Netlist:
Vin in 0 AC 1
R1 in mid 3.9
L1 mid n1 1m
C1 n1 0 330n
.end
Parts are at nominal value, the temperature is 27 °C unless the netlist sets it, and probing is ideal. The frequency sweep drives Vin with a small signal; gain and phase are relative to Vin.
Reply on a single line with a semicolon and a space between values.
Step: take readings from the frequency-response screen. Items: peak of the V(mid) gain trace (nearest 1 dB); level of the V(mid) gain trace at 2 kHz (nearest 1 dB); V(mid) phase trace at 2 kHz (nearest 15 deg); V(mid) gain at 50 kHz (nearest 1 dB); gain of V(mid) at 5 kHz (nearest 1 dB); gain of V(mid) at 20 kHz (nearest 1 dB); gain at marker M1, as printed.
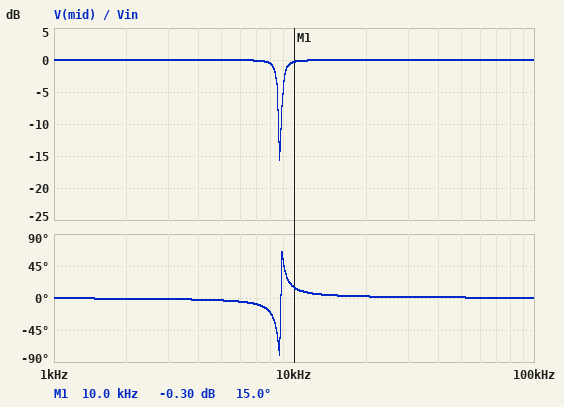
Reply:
0 dB; 0 dB; 0 deg; 0 dB; 0 dB; 0 dB; -0.30 dB
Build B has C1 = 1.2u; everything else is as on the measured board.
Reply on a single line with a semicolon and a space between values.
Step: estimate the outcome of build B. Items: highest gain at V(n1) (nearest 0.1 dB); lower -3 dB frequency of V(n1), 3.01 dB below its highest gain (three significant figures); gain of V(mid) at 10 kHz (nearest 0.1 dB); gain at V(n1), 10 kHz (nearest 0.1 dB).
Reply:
17.4 dB; 4.25 kHz; 0 dB; -11.5 dB
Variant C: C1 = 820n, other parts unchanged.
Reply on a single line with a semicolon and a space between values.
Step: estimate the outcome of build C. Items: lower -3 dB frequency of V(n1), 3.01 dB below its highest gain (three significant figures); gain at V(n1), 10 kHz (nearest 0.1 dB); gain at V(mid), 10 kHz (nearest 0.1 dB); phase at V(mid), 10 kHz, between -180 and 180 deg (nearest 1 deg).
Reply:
5.22 kHz; -7.0 dB; 0 dB; 5 deg
